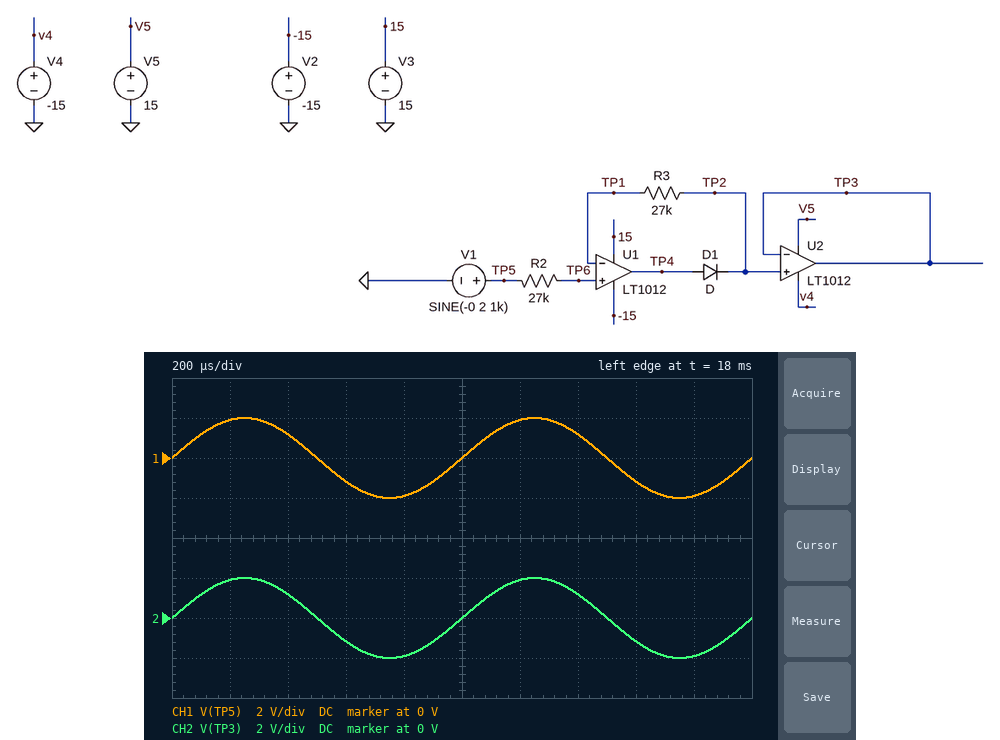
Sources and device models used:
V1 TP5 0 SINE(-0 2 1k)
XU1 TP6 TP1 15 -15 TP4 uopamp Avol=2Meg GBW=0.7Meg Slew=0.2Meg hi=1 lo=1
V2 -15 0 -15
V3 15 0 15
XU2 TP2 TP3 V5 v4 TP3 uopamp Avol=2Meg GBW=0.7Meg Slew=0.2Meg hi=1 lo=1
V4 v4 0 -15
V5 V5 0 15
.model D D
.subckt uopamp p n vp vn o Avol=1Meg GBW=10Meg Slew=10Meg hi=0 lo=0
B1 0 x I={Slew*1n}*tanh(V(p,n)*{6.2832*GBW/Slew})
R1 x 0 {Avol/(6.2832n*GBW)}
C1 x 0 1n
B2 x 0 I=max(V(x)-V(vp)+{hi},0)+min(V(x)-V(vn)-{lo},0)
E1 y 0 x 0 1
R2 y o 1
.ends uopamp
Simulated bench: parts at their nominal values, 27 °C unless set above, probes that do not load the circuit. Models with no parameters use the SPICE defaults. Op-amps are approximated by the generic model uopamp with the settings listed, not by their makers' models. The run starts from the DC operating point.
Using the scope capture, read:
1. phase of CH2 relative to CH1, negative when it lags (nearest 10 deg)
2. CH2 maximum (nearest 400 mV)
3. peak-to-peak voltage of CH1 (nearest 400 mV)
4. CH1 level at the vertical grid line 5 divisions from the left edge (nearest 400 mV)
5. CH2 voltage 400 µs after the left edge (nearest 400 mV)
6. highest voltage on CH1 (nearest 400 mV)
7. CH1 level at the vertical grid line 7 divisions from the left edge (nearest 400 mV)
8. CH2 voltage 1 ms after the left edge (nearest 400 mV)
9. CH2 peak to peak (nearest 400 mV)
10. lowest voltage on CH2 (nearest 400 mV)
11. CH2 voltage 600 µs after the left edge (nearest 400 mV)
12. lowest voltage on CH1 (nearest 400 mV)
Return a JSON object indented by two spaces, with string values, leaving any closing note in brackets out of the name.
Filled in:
{
  "phase of CH2 relative to CH1, negative when it lags": "0 deg",
  "CH2 maximum": "2.0 V",
  "peak-to-peak voltage of CH1": "4.0 V",
  "CH1 level at the vertical grid line 5 divisions from the left edge": "0 V",
  "CH2 voltage 400 µs after the left edge": "1.2 V",
  "highest voltage on CH1": "2.0 V",
  "CH1 level at the vertical grid line 7 divisions from the left edge": "1.2 V",
  "CH2 voltage 1 ms after the left edge": "0 V",
  "CH2 peak to peak": "4.0 V",
  "lowest voltage on CH2": "-2.0 V",
  "CH2 voltage 600 µs after the left edge": "-1.2 V",
  "lowest voltage on CH1": "-2.0 V"
}
